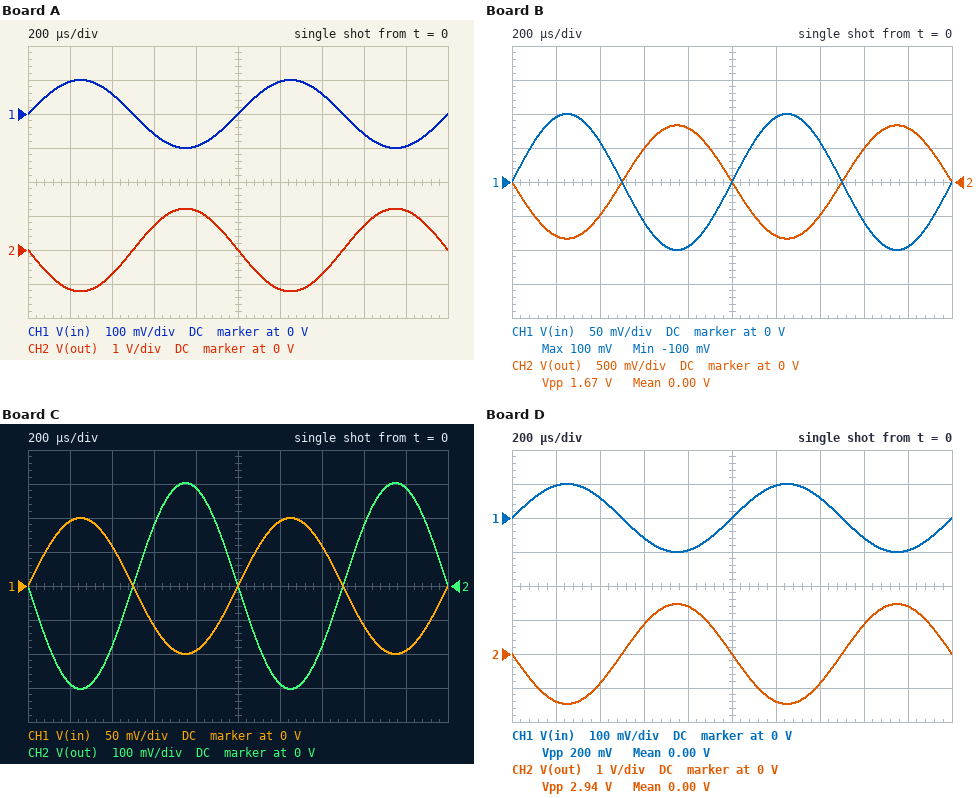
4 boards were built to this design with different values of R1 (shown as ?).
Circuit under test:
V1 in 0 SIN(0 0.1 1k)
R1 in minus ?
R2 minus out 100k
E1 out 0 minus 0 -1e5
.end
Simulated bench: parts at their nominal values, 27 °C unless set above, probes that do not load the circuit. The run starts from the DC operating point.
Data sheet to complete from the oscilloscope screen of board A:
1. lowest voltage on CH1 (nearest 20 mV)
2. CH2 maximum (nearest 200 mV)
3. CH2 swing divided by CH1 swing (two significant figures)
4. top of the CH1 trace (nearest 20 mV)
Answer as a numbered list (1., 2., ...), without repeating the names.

1. -100 mV
2. 1.2 V
3. 12
4. 100 mV
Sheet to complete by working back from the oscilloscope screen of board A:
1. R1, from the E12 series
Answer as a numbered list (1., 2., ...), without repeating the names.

1. 8.2 kΩ
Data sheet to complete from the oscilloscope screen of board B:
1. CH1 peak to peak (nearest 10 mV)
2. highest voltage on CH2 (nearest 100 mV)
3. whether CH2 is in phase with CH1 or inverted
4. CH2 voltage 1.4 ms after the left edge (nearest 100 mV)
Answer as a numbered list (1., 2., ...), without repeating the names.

1. 200 mV
2. 800 mV
3. inverted
4. -500 mV
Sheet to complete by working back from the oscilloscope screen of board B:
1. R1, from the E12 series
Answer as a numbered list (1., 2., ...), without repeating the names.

1. 12 kΩ
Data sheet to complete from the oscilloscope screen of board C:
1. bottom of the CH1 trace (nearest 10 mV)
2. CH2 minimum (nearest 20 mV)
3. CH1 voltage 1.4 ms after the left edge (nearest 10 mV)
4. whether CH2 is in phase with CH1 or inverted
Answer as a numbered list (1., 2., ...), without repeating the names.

1. -100 mV
2. -300 mV
3. 60 mV
4. inverted
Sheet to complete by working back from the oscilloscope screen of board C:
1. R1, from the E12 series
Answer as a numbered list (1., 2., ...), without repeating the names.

1. 33 kΩ
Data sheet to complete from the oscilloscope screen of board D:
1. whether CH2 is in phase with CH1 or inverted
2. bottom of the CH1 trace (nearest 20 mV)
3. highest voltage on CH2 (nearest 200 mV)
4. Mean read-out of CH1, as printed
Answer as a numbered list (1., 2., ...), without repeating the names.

1. inverted
2. -100 mV
3. 1.4 V
4. 0.00 V
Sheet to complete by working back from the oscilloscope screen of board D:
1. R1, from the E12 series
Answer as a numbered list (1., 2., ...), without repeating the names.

1. 6.8 kΩ
